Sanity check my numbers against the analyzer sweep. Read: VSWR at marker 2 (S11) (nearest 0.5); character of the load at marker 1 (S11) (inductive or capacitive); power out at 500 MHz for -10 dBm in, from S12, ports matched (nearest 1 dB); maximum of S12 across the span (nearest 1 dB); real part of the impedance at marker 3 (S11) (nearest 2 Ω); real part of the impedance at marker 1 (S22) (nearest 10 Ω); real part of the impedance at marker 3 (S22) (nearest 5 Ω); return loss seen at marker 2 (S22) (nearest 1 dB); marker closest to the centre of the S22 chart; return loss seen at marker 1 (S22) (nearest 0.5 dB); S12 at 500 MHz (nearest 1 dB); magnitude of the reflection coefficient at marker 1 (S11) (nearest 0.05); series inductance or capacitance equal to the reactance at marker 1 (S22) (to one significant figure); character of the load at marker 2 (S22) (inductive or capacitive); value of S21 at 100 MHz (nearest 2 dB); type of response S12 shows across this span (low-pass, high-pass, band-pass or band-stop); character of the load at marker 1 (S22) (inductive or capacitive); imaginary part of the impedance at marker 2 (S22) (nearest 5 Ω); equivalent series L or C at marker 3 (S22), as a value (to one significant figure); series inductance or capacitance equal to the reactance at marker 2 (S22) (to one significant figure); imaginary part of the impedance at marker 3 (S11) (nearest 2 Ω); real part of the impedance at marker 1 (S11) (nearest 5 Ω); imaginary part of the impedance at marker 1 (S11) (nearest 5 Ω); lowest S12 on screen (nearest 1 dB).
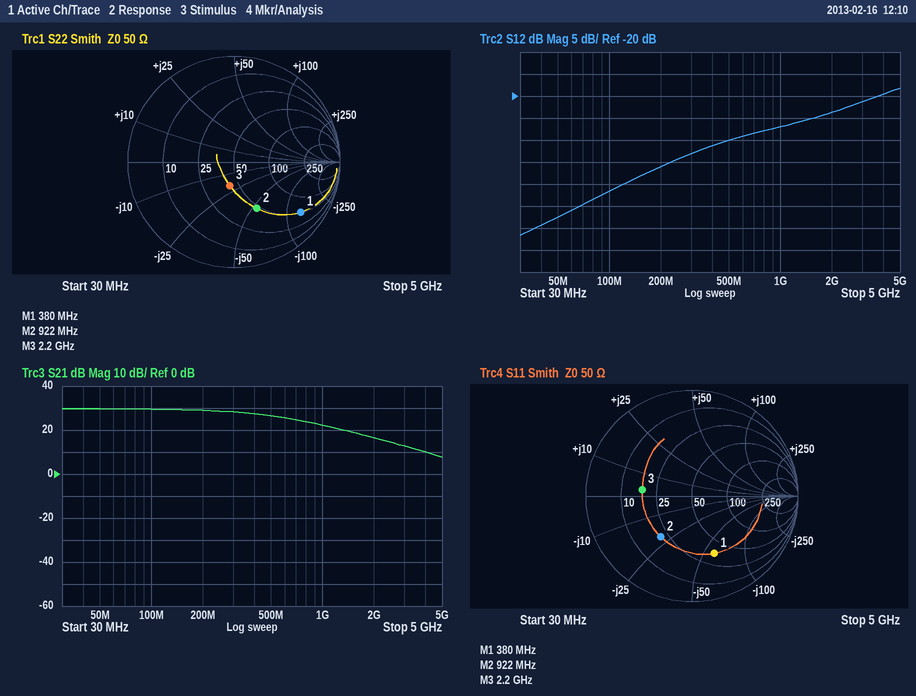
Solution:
3.0
capacitive
-40 dBm
-18 dB
18 Ω
50 Ω
40 Ω
6 dB
marker 3
2.0 dB
-30 dB
0.60
3 pF
capacitive
30 dB
high-pass
capacitive
-55 Ω
4 pF
3 pF
+2 Ω
35 Ω
-60 Ω
-52 dB
